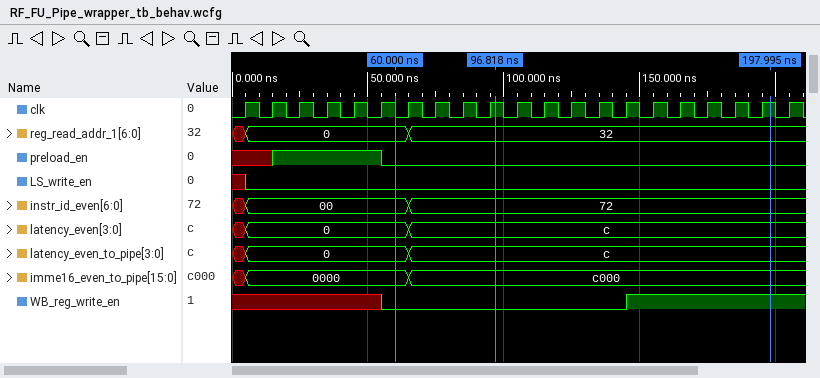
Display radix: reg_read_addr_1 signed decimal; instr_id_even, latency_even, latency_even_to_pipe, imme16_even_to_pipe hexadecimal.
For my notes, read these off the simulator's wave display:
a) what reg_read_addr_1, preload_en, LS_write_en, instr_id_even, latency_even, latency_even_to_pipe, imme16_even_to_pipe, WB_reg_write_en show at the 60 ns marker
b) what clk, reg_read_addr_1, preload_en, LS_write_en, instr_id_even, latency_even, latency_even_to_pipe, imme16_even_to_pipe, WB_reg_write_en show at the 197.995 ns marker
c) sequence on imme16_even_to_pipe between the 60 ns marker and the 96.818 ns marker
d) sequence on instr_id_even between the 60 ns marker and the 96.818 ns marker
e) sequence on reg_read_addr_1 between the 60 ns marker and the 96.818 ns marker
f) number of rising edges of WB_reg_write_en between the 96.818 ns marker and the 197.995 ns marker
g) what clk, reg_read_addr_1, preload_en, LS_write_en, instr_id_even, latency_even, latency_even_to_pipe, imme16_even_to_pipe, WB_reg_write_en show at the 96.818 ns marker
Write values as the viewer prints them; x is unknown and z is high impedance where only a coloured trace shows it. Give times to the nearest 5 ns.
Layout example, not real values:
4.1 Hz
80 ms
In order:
reg_read_addr_1=0, preload_en=0, LS_write_en=0, instr_id_even=00, latency_even=0, latency_even_to_pipe=0, imme16_even_to_pipe=0000, WB_reg_write_en=0
clk=1, reg_read_addr_1=32, preload_en=0, LS_write_en=0, instr_id_even=72, latency_even=c, latency_even_to_pipe=c, imme16_even_to_pipe=c000, WB_reg_write_en=1
0000, c000
00, 72
0, 32
1
clk=1, reg_read_addr_1=32, preload_en=0, LS_write_en=0, instr_id_even=72, latency_even=c, latency_even_to_pipe=c, imme16_even_to_pipe=c000, WB_reg_write_en=0
